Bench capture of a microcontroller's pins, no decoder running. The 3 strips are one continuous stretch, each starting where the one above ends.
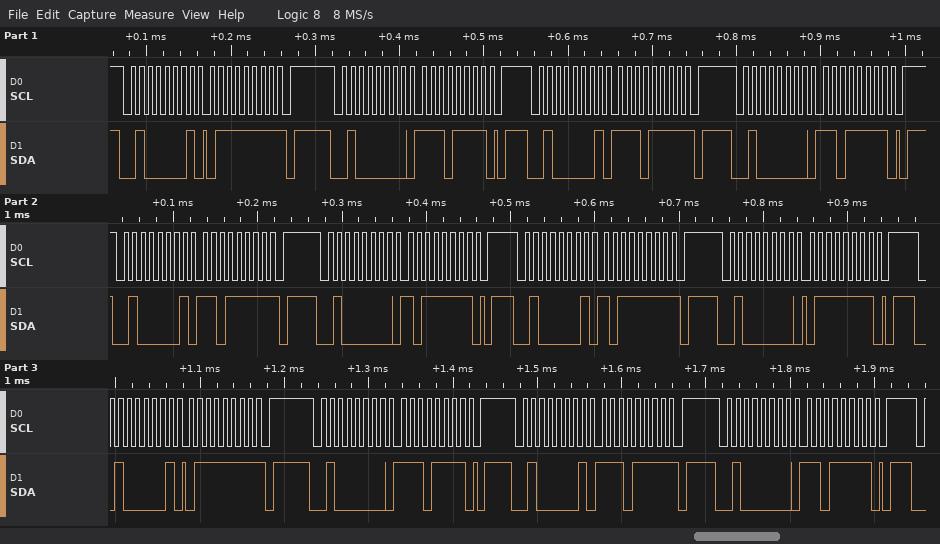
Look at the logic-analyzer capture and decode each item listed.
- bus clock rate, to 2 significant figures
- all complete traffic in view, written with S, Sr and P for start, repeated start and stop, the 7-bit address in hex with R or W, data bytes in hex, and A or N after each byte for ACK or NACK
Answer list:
100 kHz
S 20R A 7F N P S 20W A EF A P S 20R A EF N P S 20W A DF A P S 20R A DF N P S 20W A BF A P S 20R A BF N P S 20W A 7F A P S 20R A 7F N P S 20W A EF A P S 20R A EF N P S 20W A DF A P
